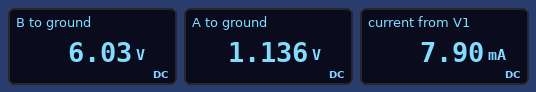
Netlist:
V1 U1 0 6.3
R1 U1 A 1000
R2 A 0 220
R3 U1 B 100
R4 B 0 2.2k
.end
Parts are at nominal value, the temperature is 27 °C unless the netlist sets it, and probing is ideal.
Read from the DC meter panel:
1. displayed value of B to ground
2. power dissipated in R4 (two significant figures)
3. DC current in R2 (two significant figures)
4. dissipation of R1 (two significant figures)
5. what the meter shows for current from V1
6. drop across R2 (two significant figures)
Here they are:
6.03 V
17 mW
5.2 mA
27 mW
7.90 mA
1.1 V
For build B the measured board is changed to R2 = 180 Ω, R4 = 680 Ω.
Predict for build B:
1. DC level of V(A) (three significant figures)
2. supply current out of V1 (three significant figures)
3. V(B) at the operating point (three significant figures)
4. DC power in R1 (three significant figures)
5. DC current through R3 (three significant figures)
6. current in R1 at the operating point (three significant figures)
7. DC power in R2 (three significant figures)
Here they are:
961 mV
13.4 mA
5.49 V
28.5 mW
8.08 mA
5.34 mA
5.13 mW
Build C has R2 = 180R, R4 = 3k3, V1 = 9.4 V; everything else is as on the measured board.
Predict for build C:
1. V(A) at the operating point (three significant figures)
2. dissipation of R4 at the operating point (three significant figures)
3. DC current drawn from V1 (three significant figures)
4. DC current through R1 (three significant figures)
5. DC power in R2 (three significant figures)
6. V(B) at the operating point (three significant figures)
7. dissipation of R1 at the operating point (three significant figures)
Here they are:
1.43 V
25.2 mW
10.7 mA
7.97 mA
11.4 mW
9.12 V
63.5 mW
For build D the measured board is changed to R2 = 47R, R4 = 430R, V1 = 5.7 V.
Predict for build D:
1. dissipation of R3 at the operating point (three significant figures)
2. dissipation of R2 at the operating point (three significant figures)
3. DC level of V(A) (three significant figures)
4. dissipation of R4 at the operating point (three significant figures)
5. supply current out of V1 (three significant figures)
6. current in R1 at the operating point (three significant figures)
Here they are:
11.6 mW
1.39 mW
256 mV
49.7 mW
16.2 mA
5.44 mA
